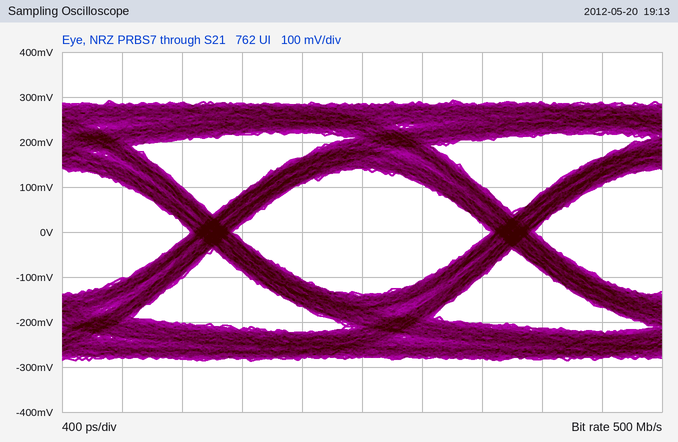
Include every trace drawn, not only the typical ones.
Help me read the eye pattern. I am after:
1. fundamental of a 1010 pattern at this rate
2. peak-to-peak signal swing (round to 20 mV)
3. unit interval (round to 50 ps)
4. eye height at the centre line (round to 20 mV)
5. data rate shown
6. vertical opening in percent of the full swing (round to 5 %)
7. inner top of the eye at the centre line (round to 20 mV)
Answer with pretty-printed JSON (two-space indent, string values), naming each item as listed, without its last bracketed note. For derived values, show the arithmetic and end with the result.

{
  "fundamental of a 1010 pattern at this rate": "250 MHz",
  "peak-to-peak signal swing": "580 mV",
  "unit interval": "2.00 ns",
  "eye height at the centre line": "280 mV",
  "data rate shown": "500 Mb/s",
  "vertical opening in percent of the full swing": "280 mV / 580 mV ≈ 48.3 %, so 50 % to the nearest 5 %",
  "inner top of the eye at the centre line": "140 mV"
}
